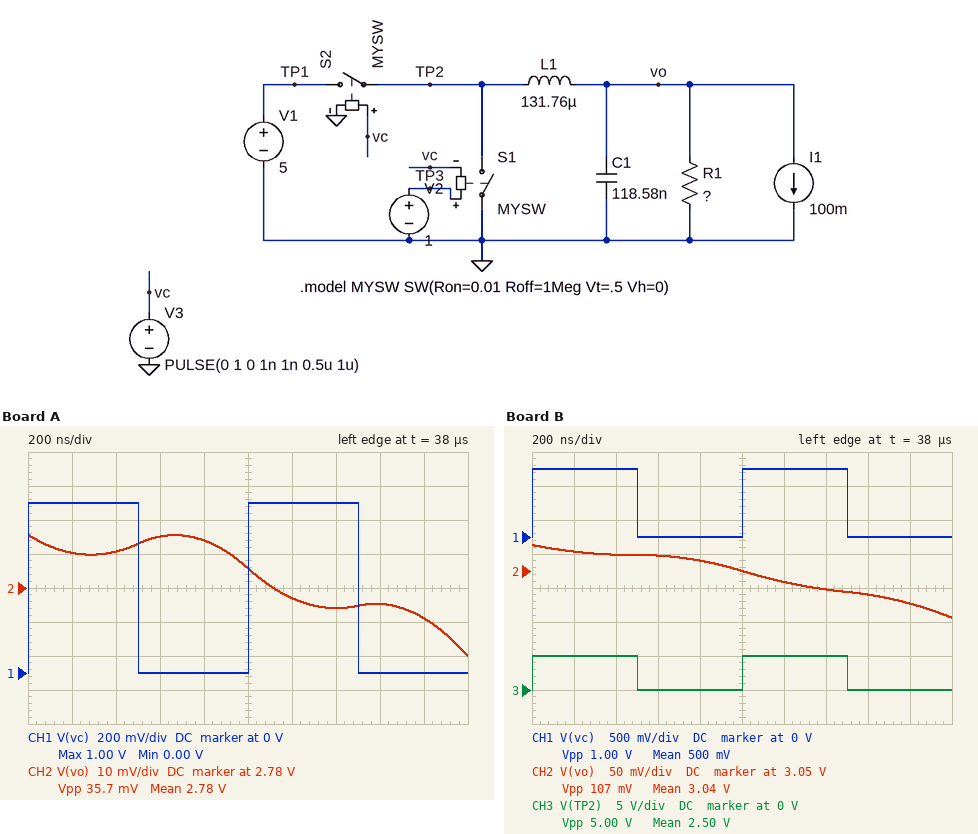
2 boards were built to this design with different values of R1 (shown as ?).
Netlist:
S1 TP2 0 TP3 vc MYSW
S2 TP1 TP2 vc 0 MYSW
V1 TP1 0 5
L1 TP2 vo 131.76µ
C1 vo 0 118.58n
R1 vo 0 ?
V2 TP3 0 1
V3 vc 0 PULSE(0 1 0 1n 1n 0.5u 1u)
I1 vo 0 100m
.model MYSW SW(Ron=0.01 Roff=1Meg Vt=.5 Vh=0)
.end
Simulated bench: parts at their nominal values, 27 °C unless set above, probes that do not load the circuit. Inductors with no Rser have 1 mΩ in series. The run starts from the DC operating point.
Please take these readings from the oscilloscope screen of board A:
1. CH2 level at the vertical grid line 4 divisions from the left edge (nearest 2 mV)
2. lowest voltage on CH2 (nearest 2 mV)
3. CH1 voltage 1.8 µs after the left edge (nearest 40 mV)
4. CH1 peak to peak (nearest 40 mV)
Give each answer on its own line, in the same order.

2.794 V
2.760 V
0 V
1.00 V
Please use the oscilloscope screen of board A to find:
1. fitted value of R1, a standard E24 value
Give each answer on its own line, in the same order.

75 Ω
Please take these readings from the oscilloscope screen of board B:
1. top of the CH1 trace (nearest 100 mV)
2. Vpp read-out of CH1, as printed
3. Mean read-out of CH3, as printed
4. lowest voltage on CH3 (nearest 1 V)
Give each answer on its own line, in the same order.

1.0 V
1.00 V
2.50 V
0 V
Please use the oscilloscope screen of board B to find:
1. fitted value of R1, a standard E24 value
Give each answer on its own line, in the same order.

110 Ω
